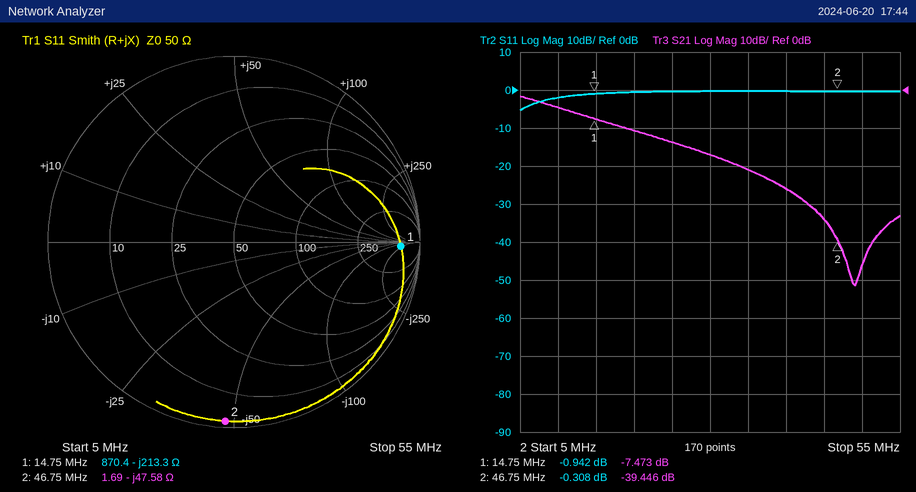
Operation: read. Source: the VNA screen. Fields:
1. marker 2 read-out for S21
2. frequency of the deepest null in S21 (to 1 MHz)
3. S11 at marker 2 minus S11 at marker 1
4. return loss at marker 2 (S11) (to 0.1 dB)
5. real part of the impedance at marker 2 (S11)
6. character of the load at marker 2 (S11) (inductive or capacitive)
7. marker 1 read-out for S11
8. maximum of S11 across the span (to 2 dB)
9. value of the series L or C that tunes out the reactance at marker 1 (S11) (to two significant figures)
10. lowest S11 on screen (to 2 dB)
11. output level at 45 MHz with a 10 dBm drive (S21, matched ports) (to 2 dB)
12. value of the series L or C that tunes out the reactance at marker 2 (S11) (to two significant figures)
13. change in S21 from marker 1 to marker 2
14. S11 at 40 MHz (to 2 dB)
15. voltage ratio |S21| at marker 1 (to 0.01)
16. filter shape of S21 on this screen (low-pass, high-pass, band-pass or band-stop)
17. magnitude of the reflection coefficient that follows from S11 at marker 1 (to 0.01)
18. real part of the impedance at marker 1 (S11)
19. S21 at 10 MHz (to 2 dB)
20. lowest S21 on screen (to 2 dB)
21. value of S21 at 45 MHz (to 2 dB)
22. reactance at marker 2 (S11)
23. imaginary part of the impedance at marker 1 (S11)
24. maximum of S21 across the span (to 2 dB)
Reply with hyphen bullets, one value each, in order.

- -39.446 dB
- 49 MHz
- 0.634 dB
- 0.3 dB
- 1.69 Ω
- capacitive
- -0.942 dB
- 0 dB
- 2.3 µH
- -6 dB
- -24 dBm
- 160 nH
- -31.973 dB
- 0 dB
- 0.42
- low-pass
- 0.90
- 870.4 Ω
- -4 dB
- -52 dB
- -34 dB
- -47.58 Ω
- -213.3 Ω
- -2 dB
